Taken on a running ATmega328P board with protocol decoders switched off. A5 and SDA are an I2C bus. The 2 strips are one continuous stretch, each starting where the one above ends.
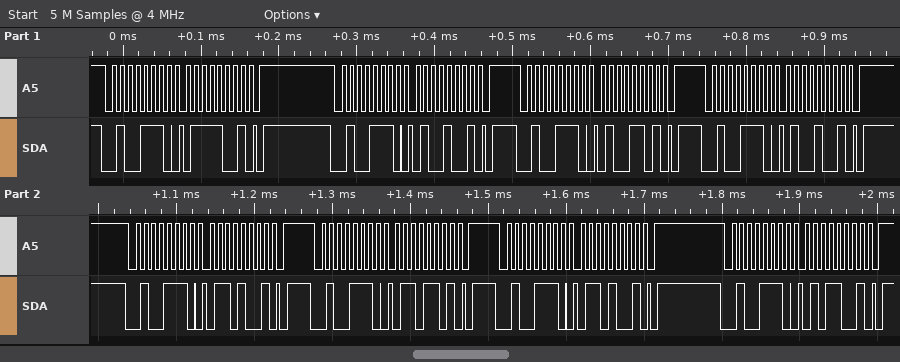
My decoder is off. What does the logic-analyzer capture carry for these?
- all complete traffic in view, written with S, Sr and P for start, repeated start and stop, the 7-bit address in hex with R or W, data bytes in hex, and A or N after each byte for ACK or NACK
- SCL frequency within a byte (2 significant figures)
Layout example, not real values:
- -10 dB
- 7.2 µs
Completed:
- S 27W A 79 A P S 27W A 49 A P S 27W A 4D A P S 27W A 49 A P S 27W A 69 A P S 27W A 6D A P S 27W A 69 A P S 27W A 59 A P
- 100 kHz
